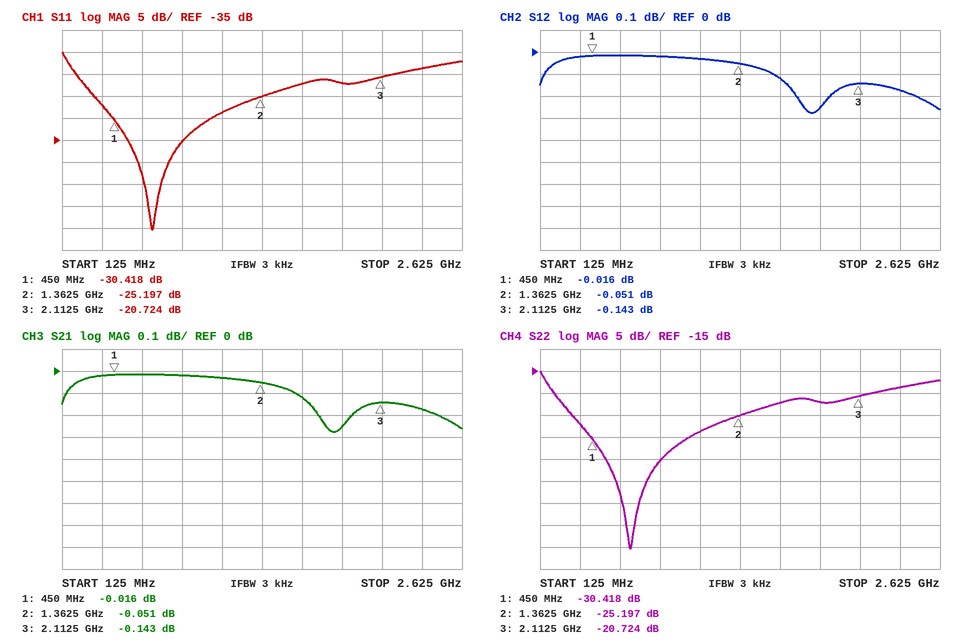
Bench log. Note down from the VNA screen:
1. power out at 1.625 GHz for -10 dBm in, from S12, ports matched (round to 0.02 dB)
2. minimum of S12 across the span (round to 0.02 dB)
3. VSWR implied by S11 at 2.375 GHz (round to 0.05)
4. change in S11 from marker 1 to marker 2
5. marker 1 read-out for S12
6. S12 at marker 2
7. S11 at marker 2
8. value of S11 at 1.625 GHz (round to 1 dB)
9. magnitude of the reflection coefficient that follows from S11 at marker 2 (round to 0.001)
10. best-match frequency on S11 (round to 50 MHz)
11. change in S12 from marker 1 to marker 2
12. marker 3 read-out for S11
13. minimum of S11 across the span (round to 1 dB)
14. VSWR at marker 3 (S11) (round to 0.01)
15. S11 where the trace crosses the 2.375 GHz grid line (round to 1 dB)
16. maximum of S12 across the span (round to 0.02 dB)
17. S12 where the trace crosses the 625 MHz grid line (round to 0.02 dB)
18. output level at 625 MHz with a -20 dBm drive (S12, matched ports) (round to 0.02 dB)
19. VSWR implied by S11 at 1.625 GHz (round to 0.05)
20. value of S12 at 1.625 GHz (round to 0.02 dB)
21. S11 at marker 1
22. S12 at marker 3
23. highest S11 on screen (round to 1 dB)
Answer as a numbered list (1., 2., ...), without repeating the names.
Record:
1. -10.12 dBm
2. -0.28 dB
3. 1.25
4. 5.221 dB
5. -0.016 dB
6. -0.051 dB
7. -25.197 dB
8. -22 dB
9. 0.055
10. 700 MHz
11. -0.035 dB
12. -20.724 dB
13. -55 dB
14. 1.20
15. -19 dB
16. -0.02 dB
17. -0.02 dB
18. -20.02 dBm
19. 1.15
20. -0.12 dB
21. -30.418 dB
22. -0.143 dB
23. -15 dB
